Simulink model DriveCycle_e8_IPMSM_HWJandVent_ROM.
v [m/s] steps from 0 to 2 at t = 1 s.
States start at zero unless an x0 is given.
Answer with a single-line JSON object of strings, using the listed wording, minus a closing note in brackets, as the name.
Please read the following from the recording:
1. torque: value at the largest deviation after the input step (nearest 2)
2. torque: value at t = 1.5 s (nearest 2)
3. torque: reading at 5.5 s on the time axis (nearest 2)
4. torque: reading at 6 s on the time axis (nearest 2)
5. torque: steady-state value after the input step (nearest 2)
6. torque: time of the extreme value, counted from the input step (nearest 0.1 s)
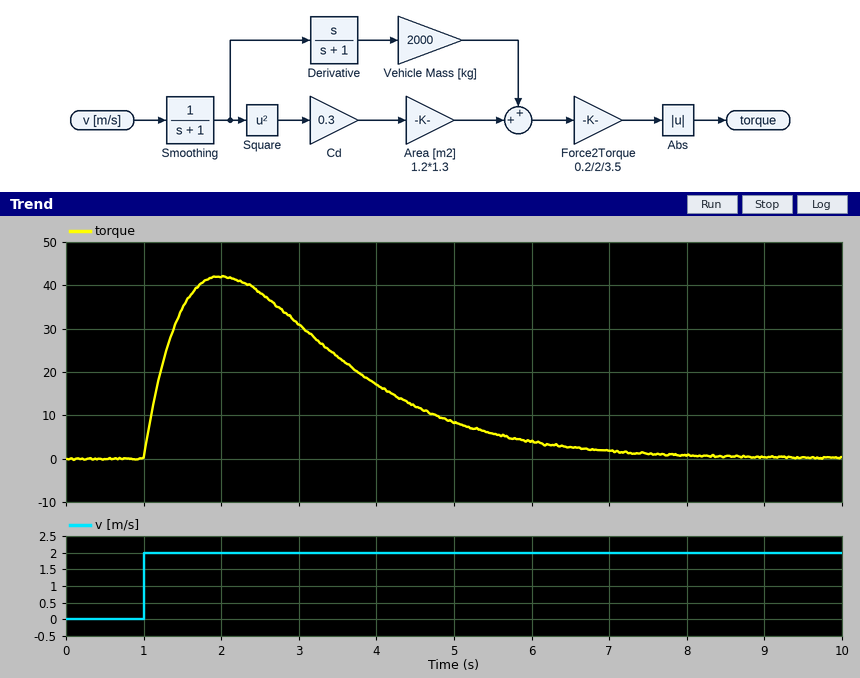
{"torque: value at the largest deviation after the input step": "42", "torque: value at t = 1.5 s": "34", "torque: reading at 5.5 s on the time axis": "6", "torque: reading at 6 s on the time axis": "4", "torque: steady-state value after the input step": "0", "torque: time of the extreme value, counted from the input step": "1.0 s"}
